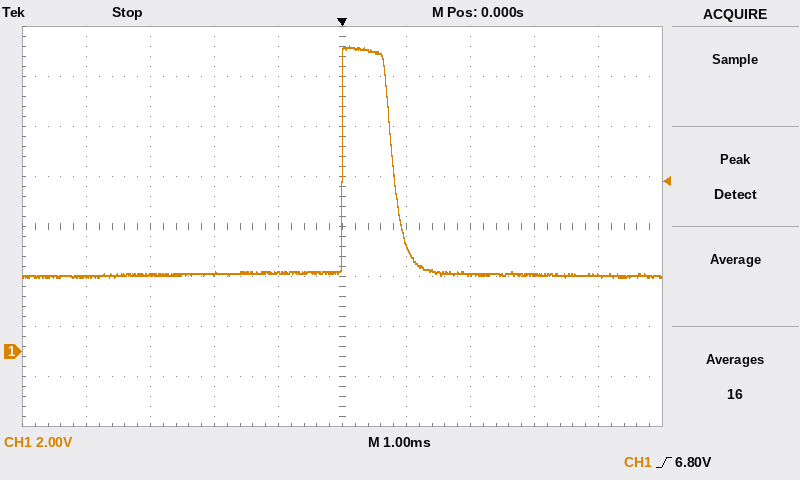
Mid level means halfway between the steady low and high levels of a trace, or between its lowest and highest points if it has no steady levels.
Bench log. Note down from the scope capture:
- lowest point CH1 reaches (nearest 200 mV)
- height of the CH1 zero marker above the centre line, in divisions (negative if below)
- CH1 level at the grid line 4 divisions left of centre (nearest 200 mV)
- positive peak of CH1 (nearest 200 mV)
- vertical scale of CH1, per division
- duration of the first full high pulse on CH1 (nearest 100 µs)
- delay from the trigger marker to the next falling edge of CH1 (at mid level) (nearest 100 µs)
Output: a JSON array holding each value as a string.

["3.0 V", "-2.5 div", "3.0 V", "12.2 V", "2 V", "800 µs", "800 µs"]
